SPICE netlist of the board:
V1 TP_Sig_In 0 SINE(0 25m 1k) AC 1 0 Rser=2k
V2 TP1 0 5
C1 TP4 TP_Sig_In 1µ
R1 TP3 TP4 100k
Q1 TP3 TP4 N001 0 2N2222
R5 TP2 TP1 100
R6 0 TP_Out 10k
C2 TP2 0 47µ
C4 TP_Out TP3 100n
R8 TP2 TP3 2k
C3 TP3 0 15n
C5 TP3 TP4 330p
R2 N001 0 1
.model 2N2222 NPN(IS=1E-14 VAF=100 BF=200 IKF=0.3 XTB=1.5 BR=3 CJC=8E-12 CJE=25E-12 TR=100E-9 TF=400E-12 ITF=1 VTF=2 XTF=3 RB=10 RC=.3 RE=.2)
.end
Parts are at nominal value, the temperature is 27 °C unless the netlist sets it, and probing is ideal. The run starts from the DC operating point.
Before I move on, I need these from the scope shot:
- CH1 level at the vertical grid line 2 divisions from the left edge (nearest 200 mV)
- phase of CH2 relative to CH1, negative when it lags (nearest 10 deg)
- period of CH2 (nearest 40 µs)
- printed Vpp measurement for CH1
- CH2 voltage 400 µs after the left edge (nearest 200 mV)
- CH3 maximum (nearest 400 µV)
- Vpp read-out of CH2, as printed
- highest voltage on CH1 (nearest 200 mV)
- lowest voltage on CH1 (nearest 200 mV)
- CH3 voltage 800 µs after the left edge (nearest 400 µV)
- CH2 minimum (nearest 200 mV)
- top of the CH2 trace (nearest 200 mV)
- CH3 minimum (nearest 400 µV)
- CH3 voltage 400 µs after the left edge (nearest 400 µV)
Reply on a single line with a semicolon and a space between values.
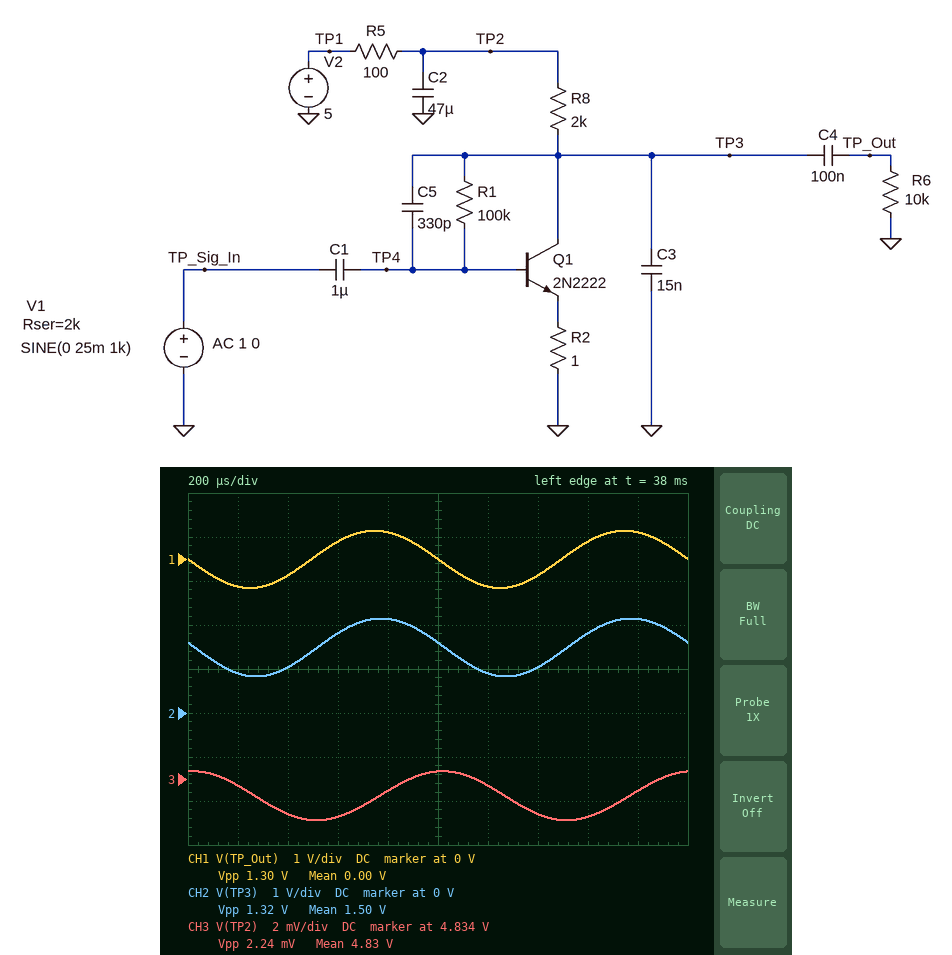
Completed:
-400 mV; -10 deg; 1.00 ms; 1.30 V; 1.0 V; 4.8344 V; 1.32 V; 600 mV; -600 mV; 4.8336 V; 800 mV; 2.2 V; 4.8320 V; 4.8324 V
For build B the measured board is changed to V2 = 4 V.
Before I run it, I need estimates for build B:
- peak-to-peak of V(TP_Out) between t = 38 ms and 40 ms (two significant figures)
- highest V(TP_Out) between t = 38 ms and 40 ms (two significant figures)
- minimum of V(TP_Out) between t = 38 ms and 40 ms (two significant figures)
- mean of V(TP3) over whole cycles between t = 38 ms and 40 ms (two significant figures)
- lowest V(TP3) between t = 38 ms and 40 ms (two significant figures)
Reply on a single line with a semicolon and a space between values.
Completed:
1.2 V; 590 mV; -620 mV; 1.3 V; 680 mV
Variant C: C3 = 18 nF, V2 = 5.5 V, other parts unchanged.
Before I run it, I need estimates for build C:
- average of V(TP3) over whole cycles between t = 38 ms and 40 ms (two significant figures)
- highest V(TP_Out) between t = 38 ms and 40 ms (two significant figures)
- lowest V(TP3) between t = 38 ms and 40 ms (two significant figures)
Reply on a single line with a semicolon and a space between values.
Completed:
1.6 V; 660 mV; 910 mV
